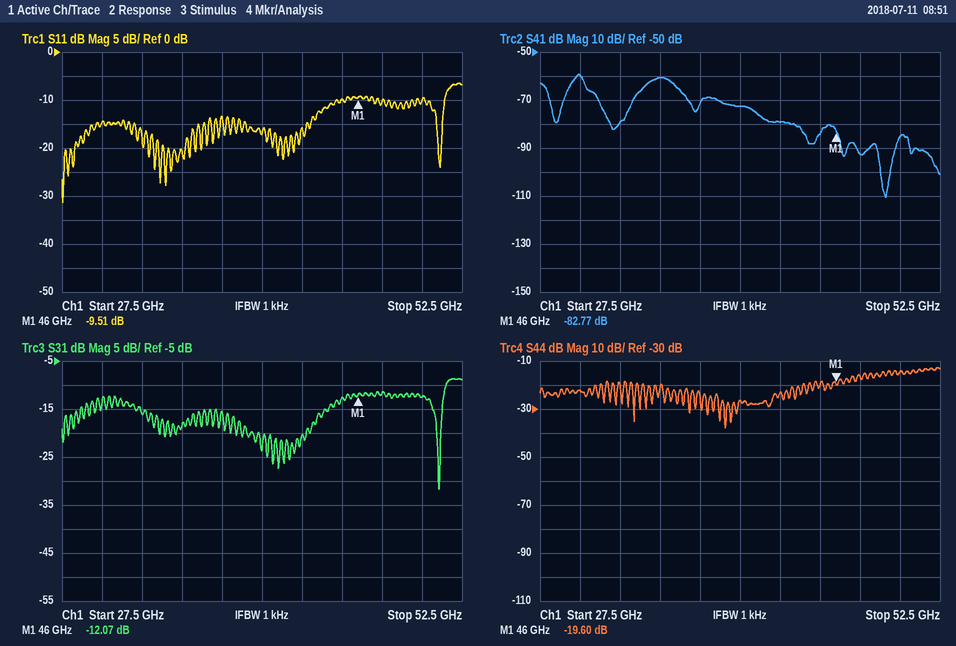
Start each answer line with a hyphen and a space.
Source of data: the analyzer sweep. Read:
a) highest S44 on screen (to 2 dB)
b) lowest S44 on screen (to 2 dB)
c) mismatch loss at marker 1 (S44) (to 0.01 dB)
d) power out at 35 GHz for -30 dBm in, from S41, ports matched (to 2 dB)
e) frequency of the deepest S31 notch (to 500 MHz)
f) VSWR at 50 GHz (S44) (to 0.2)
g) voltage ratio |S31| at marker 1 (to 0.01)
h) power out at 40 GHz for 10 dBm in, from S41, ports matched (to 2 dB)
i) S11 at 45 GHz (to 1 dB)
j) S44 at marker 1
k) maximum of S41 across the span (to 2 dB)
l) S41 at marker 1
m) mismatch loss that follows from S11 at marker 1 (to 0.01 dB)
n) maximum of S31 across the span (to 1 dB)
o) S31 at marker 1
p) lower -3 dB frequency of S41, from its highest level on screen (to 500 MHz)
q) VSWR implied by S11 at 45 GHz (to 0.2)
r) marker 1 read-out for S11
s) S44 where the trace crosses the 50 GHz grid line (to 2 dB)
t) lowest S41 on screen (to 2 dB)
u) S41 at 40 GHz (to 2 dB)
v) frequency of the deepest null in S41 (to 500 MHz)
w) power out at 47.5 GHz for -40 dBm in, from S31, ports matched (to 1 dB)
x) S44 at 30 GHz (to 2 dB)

- -12 dB
- -38 dB
- 0.05 dB
- -90 dBm
- 51.0 GHz
- 1.4
- 0.25
- -62 dBm
- -10 dB
- -19.60 dB
- -60 dB
- -82.77 dB
- 0.52 dB
- -9 dB
- -12.07 dB
- 29.5 GHz
- 2.0
- -9.51 dB
- -14 dB
- -110 dB
- -72 dB
- 49.0 GHz
- -52 dBm
- -22 dB
